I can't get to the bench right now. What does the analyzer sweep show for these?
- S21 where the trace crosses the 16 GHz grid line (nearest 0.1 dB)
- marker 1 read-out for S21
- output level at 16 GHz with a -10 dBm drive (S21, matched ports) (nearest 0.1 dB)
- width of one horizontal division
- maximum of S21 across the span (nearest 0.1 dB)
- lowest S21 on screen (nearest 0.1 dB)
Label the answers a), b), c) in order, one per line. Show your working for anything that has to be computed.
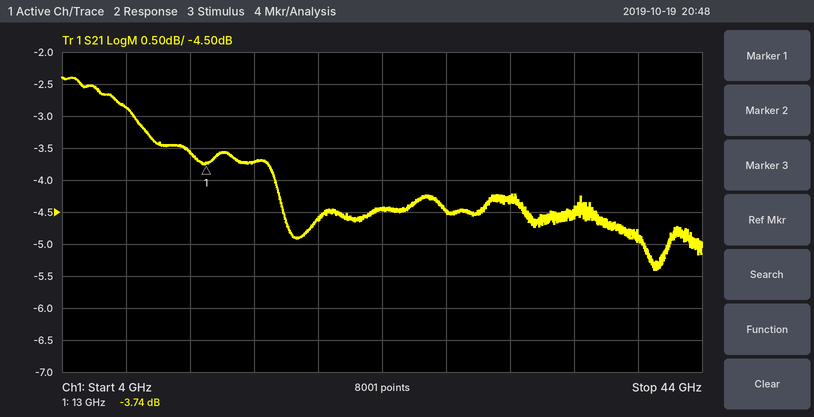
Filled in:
a) -3.7 dB
b) -3.74 dB
c) -10 dBm + (-3.7 dB) = -13.7 dBm
d) 4 GHz
e) -2.4 dB
f) -5.4 dB
